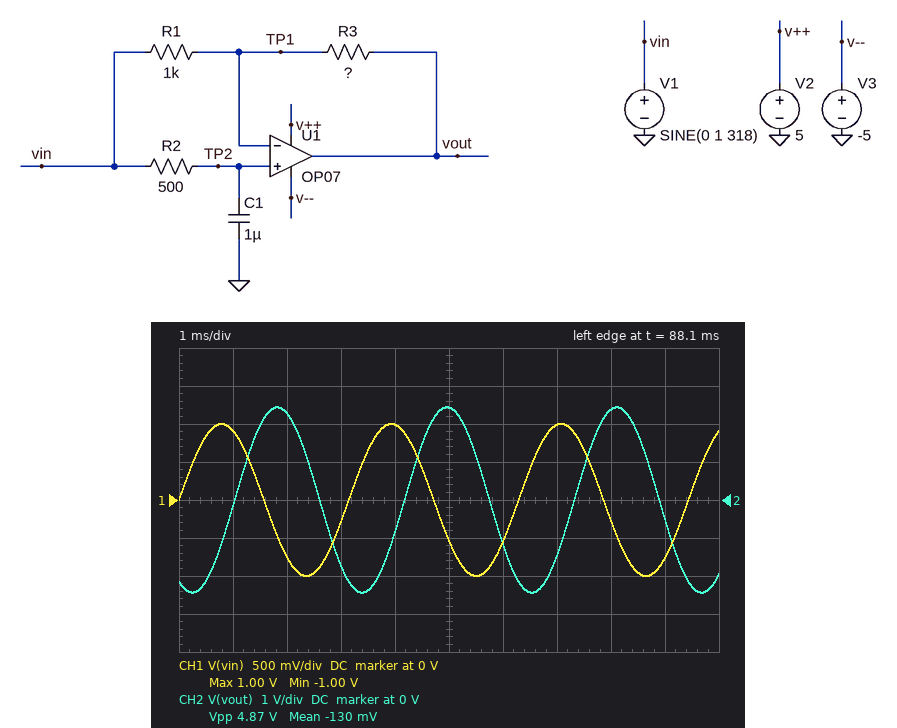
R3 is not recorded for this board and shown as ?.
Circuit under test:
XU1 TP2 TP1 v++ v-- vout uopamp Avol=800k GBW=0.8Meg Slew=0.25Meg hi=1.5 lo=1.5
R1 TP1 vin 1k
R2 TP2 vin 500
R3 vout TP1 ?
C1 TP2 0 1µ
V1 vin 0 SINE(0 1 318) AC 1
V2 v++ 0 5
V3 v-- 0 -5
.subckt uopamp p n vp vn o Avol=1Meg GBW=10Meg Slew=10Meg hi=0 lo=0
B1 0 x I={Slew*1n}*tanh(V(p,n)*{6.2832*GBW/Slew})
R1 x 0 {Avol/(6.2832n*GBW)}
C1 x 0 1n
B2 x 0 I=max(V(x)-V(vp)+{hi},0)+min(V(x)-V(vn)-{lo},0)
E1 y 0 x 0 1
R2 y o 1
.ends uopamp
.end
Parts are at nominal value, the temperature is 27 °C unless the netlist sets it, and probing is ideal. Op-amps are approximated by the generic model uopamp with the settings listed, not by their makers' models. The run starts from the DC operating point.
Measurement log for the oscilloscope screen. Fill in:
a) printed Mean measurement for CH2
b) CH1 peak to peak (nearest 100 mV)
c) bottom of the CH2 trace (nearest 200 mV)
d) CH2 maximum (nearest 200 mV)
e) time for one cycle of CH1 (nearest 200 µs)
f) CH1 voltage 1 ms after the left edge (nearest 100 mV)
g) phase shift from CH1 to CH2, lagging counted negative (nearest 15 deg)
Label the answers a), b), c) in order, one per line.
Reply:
a) -130 mV
b) 2.0 V
c) -2.4 V
d) 2.4 V
e) 3.2 ms
f) 900 mV
g) -120 deg
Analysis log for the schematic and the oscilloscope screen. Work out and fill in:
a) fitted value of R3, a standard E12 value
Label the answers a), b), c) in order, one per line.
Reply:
a) 3.3 kΩ
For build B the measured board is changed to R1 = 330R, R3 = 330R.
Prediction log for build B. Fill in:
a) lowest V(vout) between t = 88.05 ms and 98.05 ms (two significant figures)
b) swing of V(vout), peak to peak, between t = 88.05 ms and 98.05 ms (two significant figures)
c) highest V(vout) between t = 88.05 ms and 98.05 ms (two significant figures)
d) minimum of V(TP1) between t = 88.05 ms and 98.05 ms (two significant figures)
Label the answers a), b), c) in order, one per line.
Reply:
a) -1.0 V
b) 2.0 V
c) 1.0 V
d) -710 mV
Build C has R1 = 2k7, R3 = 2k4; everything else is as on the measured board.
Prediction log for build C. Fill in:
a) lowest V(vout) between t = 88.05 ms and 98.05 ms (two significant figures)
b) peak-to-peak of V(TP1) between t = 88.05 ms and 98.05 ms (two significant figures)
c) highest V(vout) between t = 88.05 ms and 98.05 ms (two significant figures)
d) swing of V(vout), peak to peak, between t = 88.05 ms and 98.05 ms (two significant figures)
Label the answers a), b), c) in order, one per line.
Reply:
a) -950 mV
b) 1.4 V
c) 950 mV
d) 1.9 V
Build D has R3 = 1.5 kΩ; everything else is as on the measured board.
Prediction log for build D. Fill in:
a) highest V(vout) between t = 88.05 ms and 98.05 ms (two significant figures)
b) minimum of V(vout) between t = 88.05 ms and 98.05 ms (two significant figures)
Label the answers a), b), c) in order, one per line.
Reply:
a) 1.3 V
b) -1.3 V
